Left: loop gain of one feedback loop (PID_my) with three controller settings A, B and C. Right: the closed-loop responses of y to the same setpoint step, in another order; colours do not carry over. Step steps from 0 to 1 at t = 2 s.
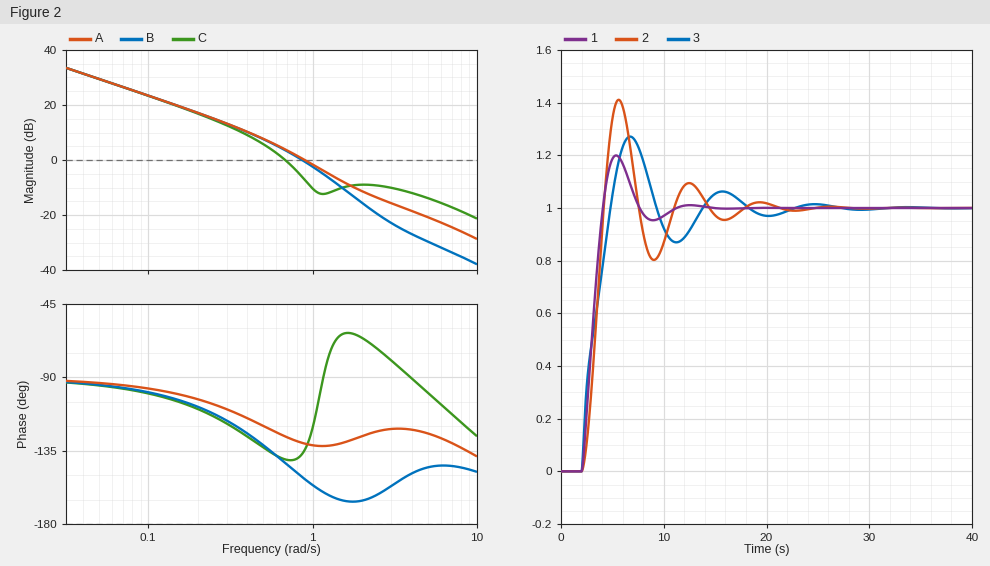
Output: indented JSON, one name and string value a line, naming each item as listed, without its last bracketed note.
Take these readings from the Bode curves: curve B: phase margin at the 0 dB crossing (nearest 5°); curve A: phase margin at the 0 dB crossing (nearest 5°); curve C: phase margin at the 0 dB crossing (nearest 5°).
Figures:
{
  "curve B: phase margin at the 0 dB crossing": "30°",
  "curve A: phase margin at the 0 dB crossing": "50°",
  "curve C: phase margin at the 0 dB crossing": "40°"
}
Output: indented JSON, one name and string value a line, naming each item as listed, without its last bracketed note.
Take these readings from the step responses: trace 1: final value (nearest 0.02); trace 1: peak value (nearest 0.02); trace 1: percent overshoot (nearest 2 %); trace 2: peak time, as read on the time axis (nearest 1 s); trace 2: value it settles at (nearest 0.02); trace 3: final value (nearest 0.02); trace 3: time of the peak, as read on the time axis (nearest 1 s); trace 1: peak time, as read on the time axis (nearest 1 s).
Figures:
{
  "trace 1: final value": "1.00",
  "trace 1: peak value": "1.20",
  "trace 1: percent overshoot": "20 %",
  "trace 2: peak time, as read on the time axis": "6 s",
  "trace 2: value it settles at": "1.00",
  "trace 3: final value": "1.00",
  "trace 3: time of the peak, as read on the time axis": "7 s",
  "trace 1: peak time, as read on the time axis": "5 s"
}
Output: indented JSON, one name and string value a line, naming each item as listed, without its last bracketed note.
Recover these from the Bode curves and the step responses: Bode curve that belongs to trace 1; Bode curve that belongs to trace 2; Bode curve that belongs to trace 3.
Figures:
{
  "Bode curve that belongs to trace 1": "A",
  "Bode curve that belongs to trace 2": "B",
  "Bode curve that belongs to trace 3": "C"
}
